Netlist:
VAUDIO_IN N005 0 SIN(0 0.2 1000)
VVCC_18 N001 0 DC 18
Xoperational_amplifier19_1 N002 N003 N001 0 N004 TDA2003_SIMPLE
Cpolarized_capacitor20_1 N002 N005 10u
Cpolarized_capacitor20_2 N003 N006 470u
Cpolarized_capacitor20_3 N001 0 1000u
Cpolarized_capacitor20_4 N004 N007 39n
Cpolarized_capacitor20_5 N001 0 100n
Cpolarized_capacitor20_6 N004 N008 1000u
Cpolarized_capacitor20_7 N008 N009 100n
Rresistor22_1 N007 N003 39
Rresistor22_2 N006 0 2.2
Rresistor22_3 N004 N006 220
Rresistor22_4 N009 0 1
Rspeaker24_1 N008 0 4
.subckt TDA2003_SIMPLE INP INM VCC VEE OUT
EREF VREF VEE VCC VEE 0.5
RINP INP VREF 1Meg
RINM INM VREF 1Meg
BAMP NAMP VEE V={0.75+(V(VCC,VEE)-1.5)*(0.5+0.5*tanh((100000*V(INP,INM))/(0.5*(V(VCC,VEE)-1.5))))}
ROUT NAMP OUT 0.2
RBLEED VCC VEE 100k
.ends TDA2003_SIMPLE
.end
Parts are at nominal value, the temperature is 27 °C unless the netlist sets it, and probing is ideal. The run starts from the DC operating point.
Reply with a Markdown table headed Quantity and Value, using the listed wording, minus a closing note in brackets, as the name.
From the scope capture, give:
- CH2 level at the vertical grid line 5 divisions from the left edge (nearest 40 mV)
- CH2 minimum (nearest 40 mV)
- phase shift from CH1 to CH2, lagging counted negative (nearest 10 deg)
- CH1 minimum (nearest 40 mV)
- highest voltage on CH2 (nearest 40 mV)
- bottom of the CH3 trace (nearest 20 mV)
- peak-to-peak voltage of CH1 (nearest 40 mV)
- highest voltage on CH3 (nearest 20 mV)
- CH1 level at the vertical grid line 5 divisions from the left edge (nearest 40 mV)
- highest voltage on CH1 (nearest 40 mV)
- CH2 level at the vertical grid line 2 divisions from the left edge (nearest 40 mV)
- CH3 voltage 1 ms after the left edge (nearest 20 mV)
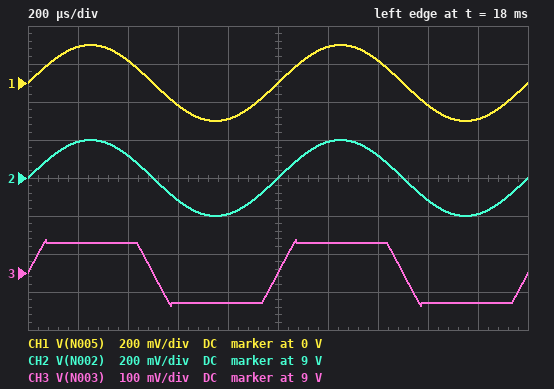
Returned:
| Quantity | Value |
|---|---|
| CH2 level at the vertical grid line 5 divisions from the left edge | 9.00 V |
| CH2 minimum | 8.80 V |
| phase shift from CH1 to CH2, lagging counted negative | 0 deg |
| CH1 minimum | -200 mV |
| highest voltage on CH2 | 9.20 V |
| bottom of the CH3 trace | 8.92 V |
| peak-to-peak voltage of CH1 | 400 mV |
| highest voltage on CH3 | 9.08 V |
| CH1 level at the vertical grid line 5 divisions from the left edge | 0 V |
| highest voltage on CH1 | 200 mV |
| CH2 level at the vertical grid line 2 divisions from the left edge | 9.12 V |
| CH3 voltage 1 ms after the left edge | 9.00 V |
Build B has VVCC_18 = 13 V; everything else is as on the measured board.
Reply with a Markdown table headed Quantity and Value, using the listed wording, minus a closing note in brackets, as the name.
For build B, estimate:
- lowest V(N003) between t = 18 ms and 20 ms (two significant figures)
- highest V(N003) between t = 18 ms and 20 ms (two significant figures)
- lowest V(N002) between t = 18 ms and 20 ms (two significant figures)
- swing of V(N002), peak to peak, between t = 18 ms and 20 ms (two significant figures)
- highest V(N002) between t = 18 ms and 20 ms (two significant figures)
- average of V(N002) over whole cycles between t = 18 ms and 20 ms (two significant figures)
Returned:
| Quantity | Value |
|---|---|
| lowest V(N003) between t = 18 ms and 20 ms | 6.4 V |
| highest V(N003) between t = 18 ms and 20 ms | 6.6 V |
| lowest V(N002) between t = 18 ms and 20 ms | 6.3 V |
| swing of V(N002), peak to peak, between t = 18 ms and 20 ms | 400 mV |
| highest V(N002) between t = 18 ms and 20 ms | 6.7 V |
| average of V(N002) over whole cycles between t = 18 ms and 20 ms | 6.5 V |
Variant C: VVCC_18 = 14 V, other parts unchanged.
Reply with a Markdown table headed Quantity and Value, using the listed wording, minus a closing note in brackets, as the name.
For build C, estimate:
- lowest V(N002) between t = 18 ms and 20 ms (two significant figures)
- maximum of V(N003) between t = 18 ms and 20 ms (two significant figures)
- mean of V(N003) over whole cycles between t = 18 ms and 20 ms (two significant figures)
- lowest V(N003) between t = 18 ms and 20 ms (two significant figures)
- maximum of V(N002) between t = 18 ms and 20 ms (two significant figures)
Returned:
| Quantity | Value |
|---|---|
| lowest V(N002) between t = 18 ms and 20 ms | 6.8 V |
| maximum of V(N003) between t = 18 ms and 20 ms | 7.1 V |
| mean of V(N003) over whole cycles between t = 18 ms and 20 ms | 7.0 V |
| lowest V(N003) between t = 18 ms and 20 ms | 6.9 V |
| maximum of V(N002) between t = 18 ms and 20 ms | 7.2 V |
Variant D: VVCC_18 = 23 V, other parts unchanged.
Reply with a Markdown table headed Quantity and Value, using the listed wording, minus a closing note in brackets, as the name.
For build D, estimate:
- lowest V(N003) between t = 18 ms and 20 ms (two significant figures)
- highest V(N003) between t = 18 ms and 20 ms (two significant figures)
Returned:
| Quantity | Value |
|---|---|
| lowest V(N003) between t = 18 ms and 20 ms | 11 V |
| highest V(N003) between t = 18 ms and 20 ms | 12 V |
